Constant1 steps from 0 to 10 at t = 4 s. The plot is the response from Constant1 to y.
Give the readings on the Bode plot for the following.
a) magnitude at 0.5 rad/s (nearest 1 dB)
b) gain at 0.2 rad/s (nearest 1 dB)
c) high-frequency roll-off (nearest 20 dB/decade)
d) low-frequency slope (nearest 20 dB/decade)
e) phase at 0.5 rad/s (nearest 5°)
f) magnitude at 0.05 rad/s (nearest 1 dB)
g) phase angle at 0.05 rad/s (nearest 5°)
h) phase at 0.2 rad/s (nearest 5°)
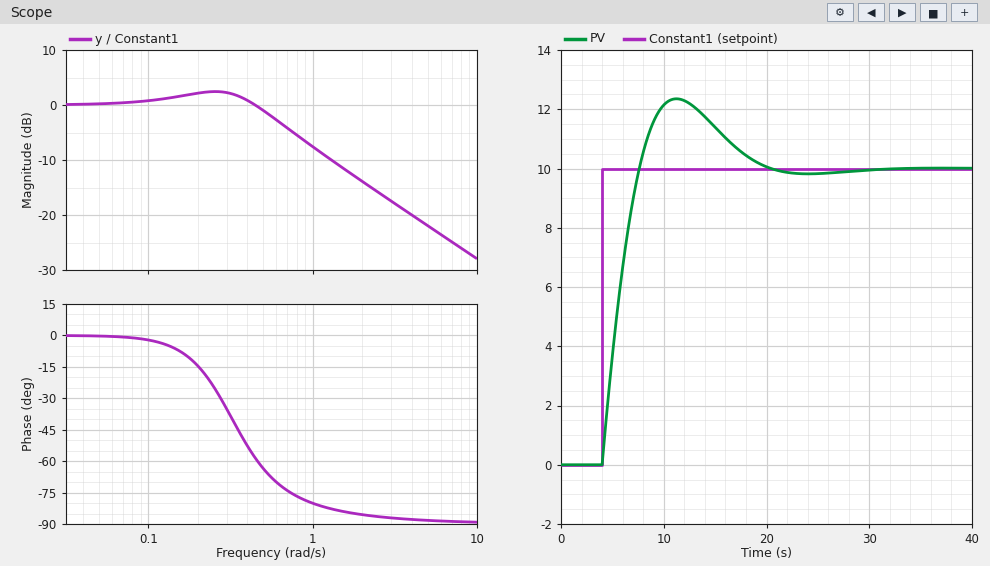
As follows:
-1 dB
2 dB
-20 dB/decade
0 dB/decade
-65°
0 dB
0°
-15°
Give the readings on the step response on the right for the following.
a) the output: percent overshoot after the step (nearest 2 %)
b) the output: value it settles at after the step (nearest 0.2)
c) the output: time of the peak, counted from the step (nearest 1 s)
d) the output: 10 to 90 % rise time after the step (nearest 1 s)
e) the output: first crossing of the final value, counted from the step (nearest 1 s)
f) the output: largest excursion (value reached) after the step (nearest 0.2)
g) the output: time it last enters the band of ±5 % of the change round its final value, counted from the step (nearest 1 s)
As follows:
24 %
10.0
7 s
3 s
4 s
12.4
14 s
